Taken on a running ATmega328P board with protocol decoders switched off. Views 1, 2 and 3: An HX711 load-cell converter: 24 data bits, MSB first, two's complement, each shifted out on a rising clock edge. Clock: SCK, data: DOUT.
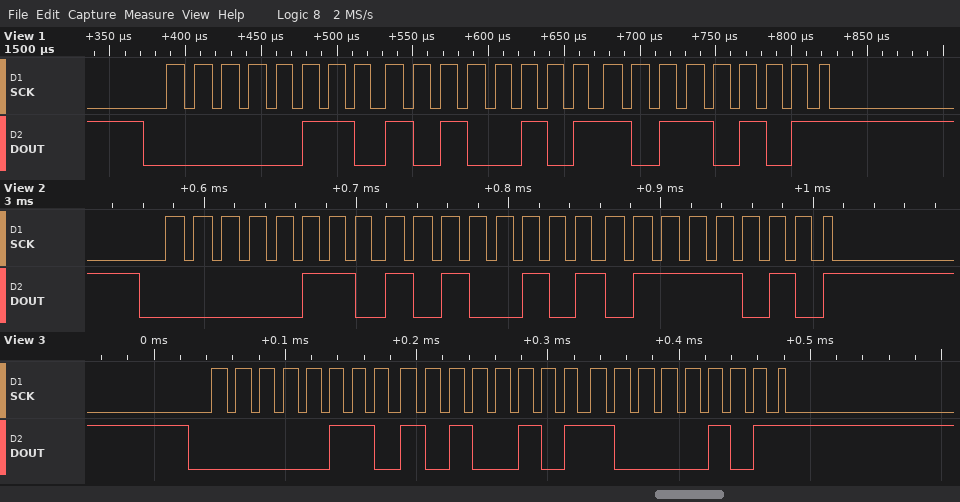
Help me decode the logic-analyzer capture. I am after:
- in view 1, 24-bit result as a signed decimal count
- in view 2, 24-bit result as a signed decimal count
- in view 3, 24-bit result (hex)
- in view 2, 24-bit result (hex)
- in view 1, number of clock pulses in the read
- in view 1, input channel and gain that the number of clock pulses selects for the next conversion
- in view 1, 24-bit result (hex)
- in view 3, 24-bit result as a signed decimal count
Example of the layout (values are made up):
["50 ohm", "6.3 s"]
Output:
["435637", "435578", "0x06A585", "0x06A57A", "25", "channel A, gain 128", "0x06A5B5", "435589"]
